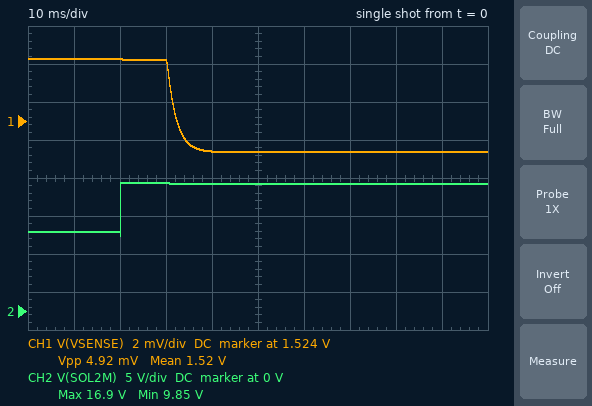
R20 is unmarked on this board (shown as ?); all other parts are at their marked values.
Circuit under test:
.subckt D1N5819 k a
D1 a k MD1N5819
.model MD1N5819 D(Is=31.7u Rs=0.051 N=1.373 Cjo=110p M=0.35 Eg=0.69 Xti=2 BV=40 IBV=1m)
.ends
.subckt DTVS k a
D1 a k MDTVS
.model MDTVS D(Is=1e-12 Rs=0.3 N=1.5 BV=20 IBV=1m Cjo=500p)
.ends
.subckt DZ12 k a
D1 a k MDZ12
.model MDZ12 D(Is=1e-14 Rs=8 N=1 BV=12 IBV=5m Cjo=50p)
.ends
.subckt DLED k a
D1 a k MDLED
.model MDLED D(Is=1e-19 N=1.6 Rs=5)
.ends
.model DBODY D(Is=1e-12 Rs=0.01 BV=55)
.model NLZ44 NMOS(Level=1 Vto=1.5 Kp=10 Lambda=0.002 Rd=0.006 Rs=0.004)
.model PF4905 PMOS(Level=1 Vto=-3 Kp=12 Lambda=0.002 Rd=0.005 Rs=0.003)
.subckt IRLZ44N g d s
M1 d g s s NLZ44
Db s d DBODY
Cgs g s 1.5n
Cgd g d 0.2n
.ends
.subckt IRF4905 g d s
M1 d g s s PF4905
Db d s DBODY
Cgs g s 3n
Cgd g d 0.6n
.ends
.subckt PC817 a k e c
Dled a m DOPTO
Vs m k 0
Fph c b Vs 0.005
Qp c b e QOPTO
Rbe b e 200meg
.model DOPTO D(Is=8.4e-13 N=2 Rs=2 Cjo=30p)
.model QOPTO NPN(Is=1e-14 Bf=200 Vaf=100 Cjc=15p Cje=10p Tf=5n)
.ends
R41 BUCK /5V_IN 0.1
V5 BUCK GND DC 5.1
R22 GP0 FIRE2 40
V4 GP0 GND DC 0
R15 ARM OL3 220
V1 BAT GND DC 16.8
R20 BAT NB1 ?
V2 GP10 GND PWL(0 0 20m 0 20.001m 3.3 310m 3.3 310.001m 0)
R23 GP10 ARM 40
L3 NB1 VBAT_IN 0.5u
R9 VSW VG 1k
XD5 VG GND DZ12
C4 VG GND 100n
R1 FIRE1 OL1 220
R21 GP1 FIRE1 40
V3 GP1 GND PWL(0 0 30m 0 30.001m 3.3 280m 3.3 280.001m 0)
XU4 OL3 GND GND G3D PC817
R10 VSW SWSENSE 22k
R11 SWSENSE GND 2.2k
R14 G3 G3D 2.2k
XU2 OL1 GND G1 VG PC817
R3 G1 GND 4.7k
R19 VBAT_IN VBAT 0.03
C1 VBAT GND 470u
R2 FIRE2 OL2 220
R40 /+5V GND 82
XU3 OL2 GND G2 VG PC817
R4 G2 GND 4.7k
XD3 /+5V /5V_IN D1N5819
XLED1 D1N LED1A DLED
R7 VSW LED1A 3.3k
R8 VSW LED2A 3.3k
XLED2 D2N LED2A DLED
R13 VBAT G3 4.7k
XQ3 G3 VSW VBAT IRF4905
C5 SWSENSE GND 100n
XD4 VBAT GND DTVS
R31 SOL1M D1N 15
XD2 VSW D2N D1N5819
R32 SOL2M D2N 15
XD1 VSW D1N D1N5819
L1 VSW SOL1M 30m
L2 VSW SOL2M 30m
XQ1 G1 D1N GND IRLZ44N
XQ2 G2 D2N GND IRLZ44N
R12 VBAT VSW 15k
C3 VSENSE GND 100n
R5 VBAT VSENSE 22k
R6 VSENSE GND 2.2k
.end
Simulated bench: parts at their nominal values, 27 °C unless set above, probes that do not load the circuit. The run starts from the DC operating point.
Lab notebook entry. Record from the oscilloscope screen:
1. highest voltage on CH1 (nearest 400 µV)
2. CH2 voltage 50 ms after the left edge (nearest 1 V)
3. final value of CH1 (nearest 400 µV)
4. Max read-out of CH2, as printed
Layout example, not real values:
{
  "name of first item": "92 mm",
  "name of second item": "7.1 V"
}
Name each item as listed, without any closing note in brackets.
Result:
{
  "highest voltage on CH1": "1.5272 V",
  "CH2 voltage 50 ms after the left edge": "17 V",
  "final value of CH1": "1.5224 V",
  "Max read-out of CH2, as printed": "16.9 V"
}
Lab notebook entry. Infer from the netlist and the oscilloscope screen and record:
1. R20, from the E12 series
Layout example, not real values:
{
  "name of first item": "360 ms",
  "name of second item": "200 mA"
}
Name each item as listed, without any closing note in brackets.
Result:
{
  "R20, from the E12 series": "0.018 Ω"
}
